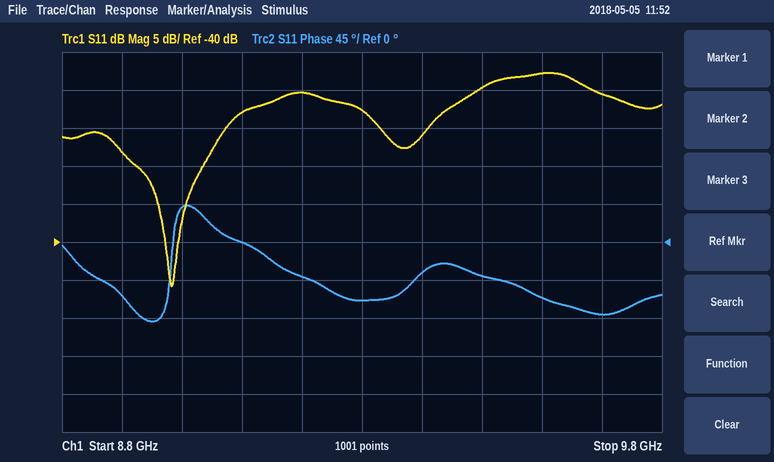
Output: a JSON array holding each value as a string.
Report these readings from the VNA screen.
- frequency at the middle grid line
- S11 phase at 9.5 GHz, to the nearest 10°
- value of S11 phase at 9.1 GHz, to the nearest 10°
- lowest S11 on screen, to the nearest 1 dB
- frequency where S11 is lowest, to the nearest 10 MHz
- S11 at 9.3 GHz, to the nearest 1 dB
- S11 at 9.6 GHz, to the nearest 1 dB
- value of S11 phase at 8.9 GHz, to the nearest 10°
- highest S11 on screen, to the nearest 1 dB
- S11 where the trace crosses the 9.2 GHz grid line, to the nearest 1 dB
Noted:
["9.3 GHz", "-40°", "0°", "-46 dB", "8.98 GHz", "-23 dB", "-18 dB", "-60°", "-18 dB", "-20 dB"]
